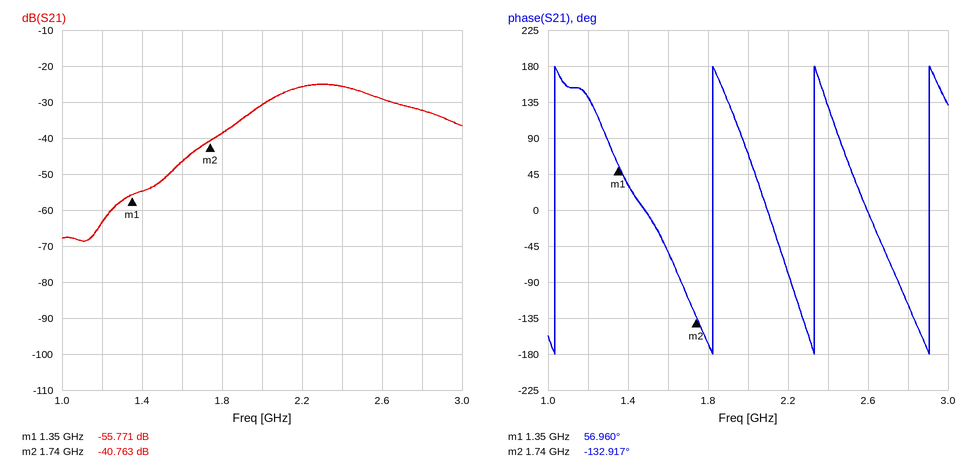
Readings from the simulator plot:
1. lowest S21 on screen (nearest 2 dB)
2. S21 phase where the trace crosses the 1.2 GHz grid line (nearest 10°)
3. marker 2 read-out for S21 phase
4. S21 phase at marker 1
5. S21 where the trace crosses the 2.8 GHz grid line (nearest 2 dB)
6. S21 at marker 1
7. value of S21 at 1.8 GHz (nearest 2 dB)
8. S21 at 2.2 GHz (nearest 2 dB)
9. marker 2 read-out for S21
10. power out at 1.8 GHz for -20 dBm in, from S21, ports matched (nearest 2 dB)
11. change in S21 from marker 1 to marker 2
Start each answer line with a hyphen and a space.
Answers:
- -68 dB
- 140°
- -132.917°
- 56.960°
- -32 dB
- -55.771 dB
- -38 dB
- -26 dB
- -40.763 dB
- -58 dBm
- 15.008 dB
